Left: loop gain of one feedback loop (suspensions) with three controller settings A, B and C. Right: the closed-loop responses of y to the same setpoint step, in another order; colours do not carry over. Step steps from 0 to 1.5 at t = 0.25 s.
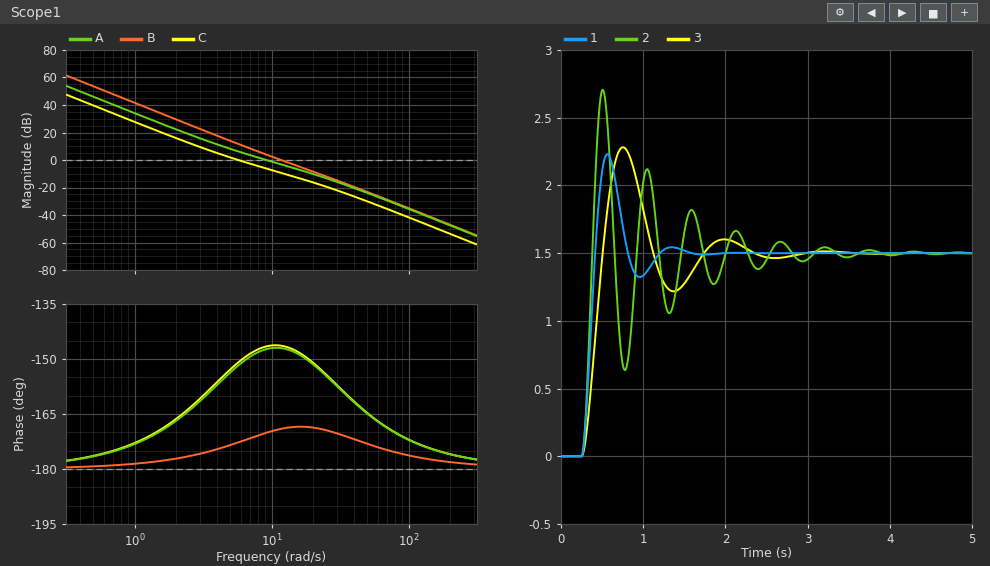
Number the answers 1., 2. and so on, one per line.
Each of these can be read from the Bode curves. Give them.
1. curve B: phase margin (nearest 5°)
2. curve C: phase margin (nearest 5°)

1. 10°
2. 30°
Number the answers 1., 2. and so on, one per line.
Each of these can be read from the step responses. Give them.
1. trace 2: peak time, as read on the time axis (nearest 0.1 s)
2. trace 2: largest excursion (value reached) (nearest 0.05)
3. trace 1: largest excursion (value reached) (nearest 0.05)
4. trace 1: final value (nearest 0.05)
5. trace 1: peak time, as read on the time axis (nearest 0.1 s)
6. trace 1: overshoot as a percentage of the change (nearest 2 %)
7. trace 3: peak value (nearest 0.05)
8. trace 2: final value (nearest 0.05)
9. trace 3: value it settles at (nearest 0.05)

1. 0.5 s
2. 2.70
3. 2.25
4. 1.50
5. 0.6 s
6. 48 %
7. 2.30
8. 1.50
9. 1.50
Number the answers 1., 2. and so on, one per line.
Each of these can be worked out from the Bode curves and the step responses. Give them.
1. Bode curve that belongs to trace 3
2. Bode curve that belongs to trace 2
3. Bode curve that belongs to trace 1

1. C
2. B
3. A
